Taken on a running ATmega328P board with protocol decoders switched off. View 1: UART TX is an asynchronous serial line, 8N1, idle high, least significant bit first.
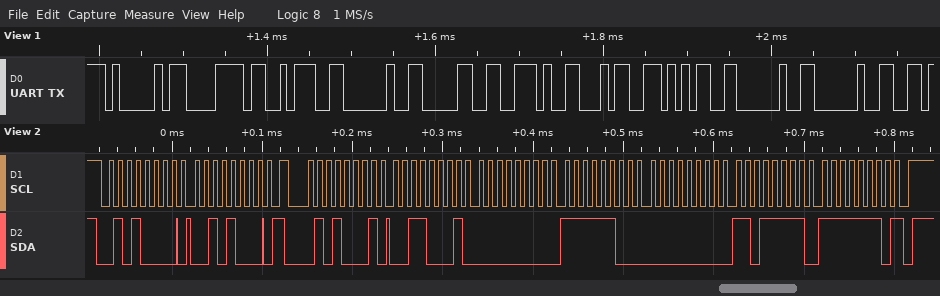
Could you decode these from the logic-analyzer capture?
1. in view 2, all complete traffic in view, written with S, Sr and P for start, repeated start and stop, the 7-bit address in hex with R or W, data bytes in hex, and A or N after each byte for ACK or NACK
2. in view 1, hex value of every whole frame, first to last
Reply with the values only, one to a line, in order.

S 28W A 28 A Sr 28R A 31 A 00 A FC A 00 A DF A FE N P
41 78 3A 20 30 2E 34 35 20 20
